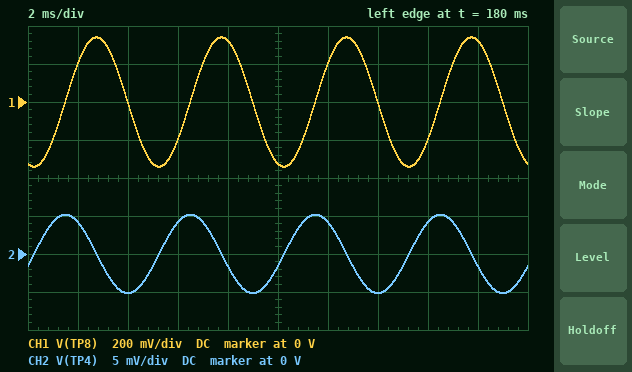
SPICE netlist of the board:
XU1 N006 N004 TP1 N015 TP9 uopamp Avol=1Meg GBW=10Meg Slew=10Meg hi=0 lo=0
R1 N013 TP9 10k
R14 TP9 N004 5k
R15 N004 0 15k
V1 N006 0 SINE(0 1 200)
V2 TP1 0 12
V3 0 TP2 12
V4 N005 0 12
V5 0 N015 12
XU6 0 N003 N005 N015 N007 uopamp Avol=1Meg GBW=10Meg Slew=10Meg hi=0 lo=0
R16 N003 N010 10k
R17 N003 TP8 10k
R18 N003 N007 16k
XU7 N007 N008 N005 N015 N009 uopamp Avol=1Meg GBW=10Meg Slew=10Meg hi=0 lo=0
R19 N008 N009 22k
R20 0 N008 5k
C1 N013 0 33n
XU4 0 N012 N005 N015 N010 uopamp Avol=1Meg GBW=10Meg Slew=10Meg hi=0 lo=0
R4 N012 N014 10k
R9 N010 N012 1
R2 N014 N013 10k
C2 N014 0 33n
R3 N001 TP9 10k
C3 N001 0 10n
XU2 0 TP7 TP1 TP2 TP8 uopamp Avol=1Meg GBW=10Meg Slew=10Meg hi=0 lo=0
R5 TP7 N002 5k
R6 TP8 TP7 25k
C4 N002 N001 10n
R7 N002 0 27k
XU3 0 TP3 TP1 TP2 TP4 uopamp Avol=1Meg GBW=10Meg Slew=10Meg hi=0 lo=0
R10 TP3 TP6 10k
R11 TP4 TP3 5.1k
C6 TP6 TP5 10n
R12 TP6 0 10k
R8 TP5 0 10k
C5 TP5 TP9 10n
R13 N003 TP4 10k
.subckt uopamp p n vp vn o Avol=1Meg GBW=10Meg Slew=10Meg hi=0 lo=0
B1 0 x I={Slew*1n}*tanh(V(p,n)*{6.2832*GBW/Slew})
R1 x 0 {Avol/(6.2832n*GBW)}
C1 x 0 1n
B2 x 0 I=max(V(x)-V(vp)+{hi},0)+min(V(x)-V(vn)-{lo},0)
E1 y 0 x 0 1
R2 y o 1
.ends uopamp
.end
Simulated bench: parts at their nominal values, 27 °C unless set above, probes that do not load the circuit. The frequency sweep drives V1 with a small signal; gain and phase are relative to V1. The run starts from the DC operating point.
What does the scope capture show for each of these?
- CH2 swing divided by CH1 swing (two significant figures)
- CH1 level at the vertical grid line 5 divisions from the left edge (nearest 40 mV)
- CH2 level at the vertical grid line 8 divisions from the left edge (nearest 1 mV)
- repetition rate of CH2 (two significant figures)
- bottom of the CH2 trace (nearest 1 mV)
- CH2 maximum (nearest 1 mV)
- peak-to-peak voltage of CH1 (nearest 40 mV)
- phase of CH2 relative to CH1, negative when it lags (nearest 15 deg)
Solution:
0.015
-320 mV
4 mV
200 Hz
-5 mV
5 mV
680 mV
90 deg
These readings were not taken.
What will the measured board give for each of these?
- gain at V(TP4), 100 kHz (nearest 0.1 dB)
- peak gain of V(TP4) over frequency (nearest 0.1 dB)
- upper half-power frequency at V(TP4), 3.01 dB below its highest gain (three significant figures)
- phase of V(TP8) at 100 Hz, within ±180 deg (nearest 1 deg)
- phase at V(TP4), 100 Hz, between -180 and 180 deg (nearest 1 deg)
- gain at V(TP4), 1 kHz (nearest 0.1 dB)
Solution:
-3.4 dB
-3.4 dB
4.53 MHz
-99 deg
-9 deg
-22.4 dB
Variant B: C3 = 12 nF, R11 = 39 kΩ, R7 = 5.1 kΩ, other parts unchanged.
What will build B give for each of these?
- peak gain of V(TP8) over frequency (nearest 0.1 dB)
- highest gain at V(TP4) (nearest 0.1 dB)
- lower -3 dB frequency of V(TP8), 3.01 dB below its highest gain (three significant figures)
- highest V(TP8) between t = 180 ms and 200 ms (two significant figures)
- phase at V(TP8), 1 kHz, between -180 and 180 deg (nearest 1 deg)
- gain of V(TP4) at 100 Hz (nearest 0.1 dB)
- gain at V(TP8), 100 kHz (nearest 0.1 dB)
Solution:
-3.3 dB
14.3 dB
619 Hz
200 mV
-150 deg
-39.9 dB
-21.1 dB
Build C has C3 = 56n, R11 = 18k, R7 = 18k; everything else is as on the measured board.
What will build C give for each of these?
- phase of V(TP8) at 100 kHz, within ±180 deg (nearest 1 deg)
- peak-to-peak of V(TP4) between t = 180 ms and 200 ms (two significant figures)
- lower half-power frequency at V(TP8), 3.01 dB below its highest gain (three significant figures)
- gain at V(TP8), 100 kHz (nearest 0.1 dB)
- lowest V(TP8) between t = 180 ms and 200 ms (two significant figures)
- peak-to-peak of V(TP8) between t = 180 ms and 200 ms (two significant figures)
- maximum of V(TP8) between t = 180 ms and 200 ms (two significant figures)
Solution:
89 deg
36 mV
218 Hz
-34.5 dB
-250 mV
500 mV
250 mV
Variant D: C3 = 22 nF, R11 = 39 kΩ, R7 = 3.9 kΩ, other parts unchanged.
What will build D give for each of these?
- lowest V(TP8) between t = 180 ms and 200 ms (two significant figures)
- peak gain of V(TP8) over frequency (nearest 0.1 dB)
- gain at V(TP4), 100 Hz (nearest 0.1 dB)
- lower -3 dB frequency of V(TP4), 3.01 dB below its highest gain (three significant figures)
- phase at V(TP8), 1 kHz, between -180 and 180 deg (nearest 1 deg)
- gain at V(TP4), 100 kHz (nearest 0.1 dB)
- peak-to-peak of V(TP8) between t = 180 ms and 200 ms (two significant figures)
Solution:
-170 mV
-7.4 dB
-39.9 dB
7.28 kHz
-159 deg
14.3 dB
340 mV
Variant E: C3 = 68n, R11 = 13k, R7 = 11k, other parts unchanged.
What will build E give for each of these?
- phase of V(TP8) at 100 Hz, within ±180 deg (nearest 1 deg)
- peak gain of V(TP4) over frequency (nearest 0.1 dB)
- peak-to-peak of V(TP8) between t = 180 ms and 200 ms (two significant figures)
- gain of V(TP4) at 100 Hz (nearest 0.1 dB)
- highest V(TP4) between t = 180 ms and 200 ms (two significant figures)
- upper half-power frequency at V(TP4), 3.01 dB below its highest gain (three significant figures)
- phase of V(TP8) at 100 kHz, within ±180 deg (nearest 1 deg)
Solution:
-117 deg
4.8 dB
410 mV
-49.4 dB
13 mV
3.50 MHz
89 deg
